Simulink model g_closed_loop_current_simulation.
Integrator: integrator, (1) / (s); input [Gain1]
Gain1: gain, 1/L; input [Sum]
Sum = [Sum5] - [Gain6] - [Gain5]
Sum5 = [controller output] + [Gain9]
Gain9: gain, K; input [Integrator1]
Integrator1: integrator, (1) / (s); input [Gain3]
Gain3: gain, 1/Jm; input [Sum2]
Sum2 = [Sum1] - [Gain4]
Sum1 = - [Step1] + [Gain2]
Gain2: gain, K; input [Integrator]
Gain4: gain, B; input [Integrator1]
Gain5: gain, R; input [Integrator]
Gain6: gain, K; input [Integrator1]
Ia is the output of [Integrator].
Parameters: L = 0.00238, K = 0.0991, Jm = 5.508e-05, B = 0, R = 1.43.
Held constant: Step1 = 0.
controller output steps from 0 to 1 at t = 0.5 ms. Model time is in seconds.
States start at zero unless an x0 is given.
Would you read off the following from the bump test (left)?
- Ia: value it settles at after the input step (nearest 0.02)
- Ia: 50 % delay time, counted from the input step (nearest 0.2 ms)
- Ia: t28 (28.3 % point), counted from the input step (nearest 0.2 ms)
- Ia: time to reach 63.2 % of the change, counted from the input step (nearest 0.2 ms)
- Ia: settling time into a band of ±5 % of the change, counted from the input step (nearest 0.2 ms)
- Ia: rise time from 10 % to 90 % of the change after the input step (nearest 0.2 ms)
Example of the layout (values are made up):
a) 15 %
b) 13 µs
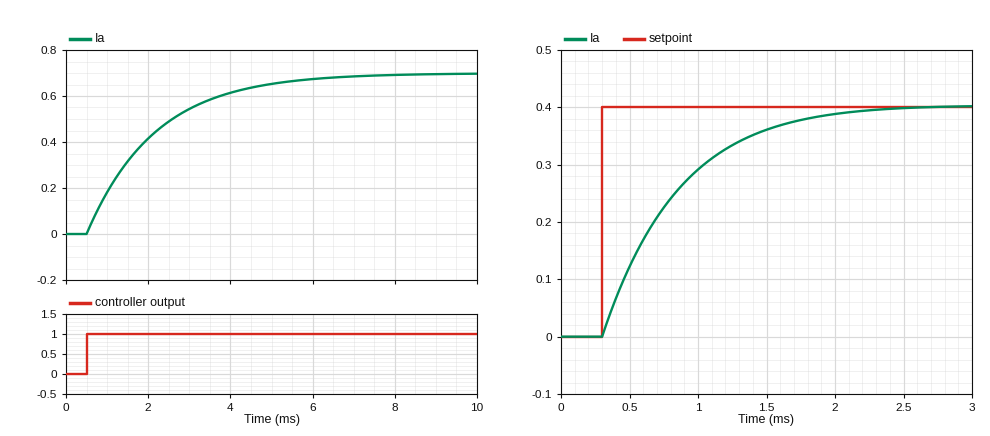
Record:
a) 0.70
b) 1.2 ms
c) 0.6 ms
d) 1.6 ms
e) 5.0 ms
f) 3.6 ms
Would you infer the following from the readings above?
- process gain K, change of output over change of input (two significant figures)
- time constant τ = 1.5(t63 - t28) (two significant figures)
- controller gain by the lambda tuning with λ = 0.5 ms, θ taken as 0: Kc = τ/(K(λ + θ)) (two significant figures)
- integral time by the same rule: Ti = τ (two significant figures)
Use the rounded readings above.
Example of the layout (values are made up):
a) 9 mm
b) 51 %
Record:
a) 0.70
b) 1.5 ms
c) 4.3
d) 1.5 ms
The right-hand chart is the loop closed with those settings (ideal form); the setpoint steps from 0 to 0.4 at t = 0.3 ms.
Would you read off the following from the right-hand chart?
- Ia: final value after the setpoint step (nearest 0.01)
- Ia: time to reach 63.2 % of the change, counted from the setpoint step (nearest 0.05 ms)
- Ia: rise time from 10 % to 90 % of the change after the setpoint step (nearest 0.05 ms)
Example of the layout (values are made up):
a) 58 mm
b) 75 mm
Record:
a) 0.40
b) 0.55 ms
c) 1.15 ms
